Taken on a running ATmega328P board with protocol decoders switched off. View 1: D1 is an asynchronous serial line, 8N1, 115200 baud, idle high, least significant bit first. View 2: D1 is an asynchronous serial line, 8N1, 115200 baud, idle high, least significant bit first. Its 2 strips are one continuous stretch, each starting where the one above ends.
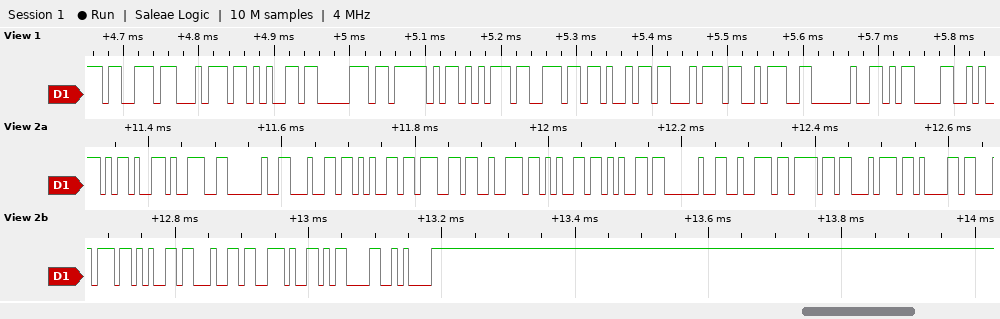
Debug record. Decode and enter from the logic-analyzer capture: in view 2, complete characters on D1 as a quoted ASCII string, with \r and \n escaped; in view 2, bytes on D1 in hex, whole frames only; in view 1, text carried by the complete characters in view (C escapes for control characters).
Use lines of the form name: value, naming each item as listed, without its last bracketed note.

in view 2, complete characters on D1 as a quoted ASCII string, with \r and \n escaped: "-9 degree rotated.\r\n"
in view 2, bytes on D1 in hex, whole frames only: 2D 39 20 64 65 67 72 65 65 20 72 6F 74 61 74 65 64 2E 0D 0A
in view 1, text carried by the complete characters in view: "step_unit: \r"
